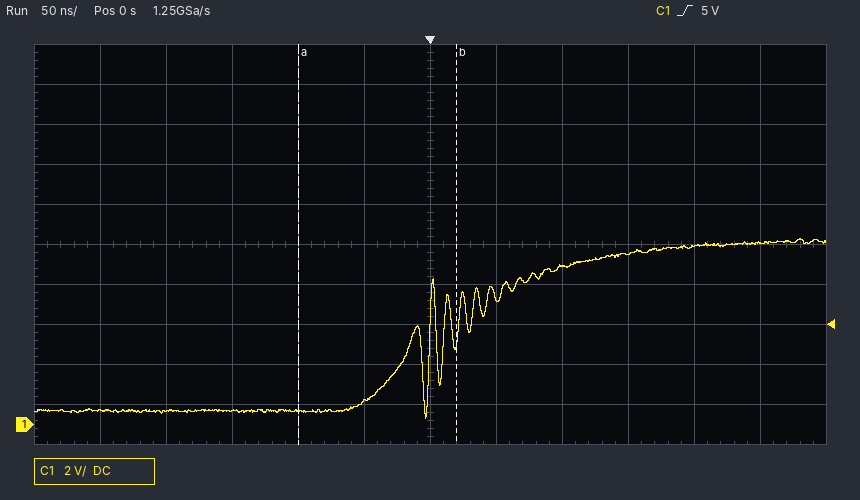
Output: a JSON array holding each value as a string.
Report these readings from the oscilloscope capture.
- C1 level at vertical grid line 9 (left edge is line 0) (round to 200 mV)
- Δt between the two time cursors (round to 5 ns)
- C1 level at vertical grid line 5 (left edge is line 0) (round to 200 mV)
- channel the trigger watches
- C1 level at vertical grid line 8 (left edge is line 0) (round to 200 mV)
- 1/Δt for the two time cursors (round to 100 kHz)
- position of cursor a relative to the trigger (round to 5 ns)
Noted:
["8.6 V", "120 ns", "1.2 V", "C1", "8.0 V", "8.3 MHz", "-100 ns"]
